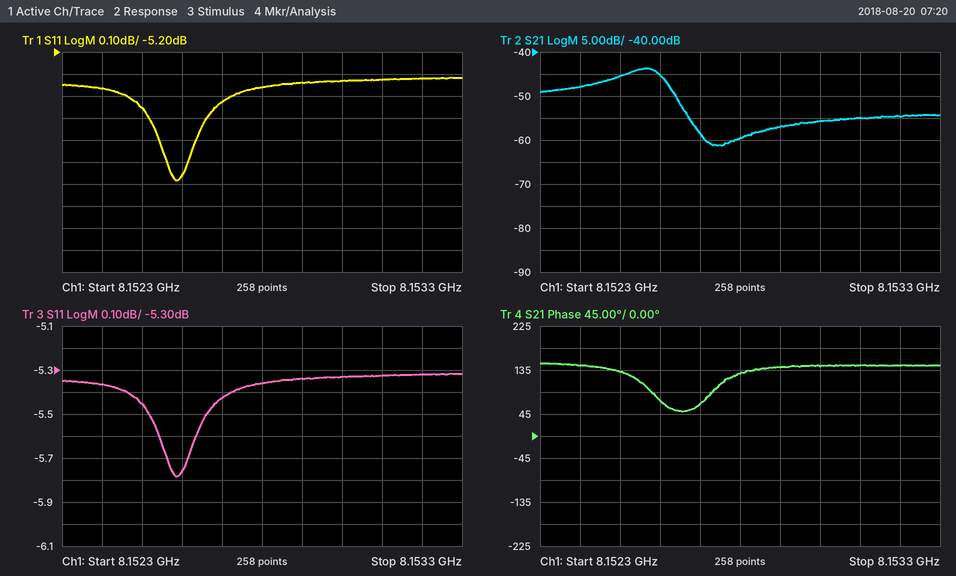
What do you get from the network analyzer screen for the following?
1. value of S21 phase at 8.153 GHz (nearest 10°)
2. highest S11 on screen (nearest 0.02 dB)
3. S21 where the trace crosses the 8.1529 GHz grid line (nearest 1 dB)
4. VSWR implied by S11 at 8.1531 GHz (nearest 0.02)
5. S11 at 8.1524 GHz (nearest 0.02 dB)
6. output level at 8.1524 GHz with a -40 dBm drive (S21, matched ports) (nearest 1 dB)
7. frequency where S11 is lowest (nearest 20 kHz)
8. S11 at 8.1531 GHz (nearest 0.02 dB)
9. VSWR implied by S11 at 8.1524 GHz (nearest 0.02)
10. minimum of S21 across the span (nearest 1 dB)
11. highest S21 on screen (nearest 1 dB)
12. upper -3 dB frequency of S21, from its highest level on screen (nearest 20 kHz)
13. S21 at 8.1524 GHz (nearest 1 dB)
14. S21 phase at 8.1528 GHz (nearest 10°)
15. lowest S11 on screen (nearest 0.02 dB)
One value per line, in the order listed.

140°
-5.32 dB
-57 dB
3.36
-5.36 dB
-88 dBm
8.15258 GHz
-5.32 dB
3.34
-61 dB
-44 dB
8.15262 GHz
-48 dB
130°
-5.78 dB
